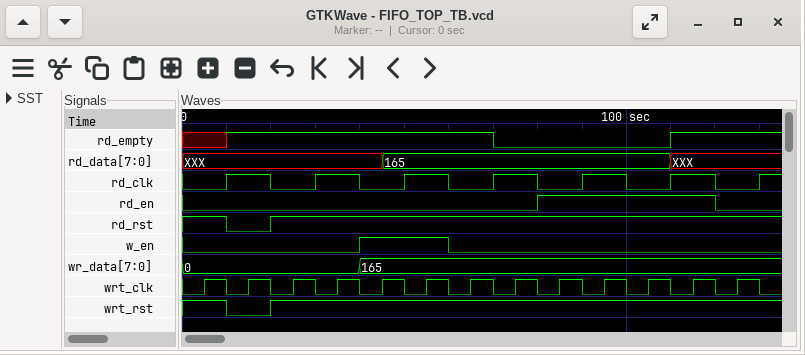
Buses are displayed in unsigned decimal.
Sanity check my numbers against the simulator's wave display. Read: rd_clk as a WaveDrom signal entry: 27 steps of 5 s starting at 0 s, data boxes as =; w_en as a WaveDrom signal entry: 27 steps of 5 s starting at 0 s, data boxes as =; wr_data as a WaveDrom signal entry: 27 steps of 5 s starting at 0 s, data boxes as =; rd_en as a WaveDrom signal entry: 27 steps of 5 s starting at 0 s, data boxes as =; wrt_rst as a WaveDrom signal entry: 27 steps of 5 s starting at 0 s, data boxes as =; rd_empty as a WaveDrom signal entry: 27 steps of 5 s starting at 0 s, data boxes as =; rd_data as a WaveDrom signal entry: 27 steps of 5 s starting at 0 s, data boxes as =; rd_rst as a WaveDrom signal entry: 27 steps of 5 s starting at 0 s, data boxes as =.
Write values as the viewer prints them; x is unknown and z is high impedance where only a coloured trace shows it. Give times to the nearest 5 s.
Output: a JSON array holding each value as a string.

["{name: 'rd_clk', wave: '0.1.0.1.0.1.0.1.0.1.0.1.0.1'}", "{name: 'w_en', wave: '0.......1...0..............'}", "{name: 'wr_data', wave: '=.......=..................', data: '0 165'}", "{name: 'rd_en', wave: '0...............1.......0..'}", "{name: 'wrt_rst', wave: '1.0.1......................'}", "{name: 'rd_empty', wave: 'x.1...........0.......1....'}", "{name: 'rd_data', wave: 'x........=............x....', data: '165'}", "{name: 'rd_rst', wave: '1.0.1......................'}"]
